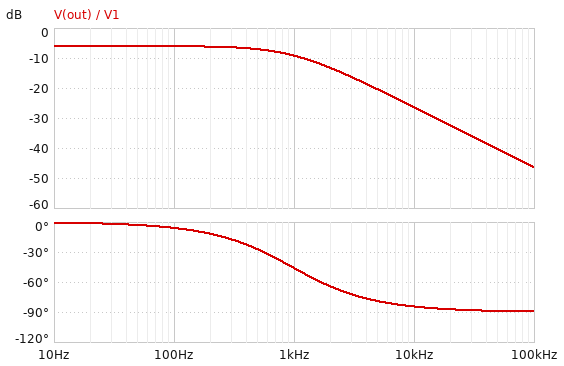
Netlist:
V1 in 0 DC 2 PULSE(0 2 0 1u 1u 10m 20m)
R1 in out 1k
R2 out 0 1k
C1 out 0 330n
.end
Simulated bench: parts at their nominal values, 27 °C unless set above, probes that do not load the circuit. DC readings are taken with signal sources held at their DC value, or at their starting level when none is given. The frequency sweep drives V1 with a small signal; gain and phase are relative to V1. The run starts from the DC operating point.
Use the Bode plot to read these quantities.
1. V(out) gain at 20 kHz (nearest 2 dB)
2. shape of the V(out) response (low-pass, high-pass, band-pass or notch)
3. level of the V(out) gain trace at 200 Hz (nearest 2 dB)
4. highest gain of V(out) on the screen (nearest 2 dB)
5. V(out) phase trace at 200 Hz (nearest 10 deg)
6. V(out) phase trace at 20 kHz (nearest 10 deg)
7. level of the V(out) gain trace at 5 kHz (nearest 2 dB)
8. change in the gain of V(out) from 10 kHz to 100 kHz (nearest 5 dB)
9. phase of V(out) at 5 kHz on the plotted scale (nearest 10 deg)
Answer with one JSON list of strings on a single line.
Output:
["-32 dB", "low-pass", "-6 dB", "-6 dB", "-10 deg", "-90 deg", "-20 dB", "-20 dB", "-80 deg"]
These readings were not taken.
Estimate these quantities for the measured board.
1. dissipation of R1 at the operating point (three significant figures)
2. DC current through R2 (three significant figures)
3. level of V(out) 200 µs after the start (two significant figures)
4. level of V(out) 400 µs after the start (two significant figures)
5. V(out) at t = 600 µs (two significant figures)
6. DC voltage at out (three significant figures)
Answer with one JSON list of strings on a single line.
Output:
["1.00 mW", "1.00 mA", "700 mV", "910 mV", "970 mV", "1.00 V"]
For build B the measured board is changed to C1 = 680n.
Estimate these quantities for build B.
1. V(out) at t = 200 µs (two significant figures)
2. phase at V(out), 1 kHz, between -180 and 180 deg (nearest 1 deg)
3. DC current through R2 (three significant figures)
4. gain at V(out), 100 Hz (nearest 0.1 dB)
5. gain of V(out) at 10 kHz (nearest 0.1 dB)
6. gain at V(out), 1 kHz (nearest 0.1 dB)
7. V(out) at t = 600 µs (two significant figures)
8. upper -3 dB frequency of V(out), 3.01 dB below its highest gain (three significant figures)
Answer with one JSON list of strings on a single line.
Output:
["440 mV", "-65 deg", "1.00 mA", "-6.2 dB", "-32.6 dB", "-13.5 dB", "830 mV", "468 Hz"]
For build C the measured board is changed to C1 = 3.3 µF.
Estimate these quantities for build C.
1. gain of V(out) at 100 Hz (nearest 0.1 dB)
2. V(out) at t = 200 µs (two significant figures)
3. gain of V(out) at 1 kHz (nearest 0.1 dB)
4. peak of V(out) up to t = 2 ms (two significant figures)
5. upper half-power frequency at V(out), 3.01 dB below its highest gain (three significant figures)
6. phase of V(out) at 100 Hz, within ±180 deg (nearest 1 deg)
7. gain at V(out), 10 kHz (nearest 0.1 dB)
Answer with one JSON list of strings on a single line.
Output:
["-9.2 dB", "110 mV", "-26.4 dB", "700 mV", "96.5 Hz", "-46 deg", "-46.3 dB"]
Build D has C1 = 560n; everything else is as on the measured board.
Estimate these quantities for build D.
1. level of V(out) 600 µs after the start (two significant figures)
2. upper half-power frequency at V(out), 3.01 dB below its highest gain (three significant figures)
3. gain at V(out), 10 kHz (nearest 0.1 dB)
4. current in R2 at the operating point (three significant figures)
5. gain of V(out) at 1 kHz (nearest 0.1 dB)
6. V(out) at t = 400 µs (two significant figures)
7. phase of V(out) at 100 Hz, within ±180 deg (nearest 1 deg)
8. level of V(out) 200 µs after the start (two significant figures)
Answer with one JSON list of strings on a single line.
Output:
["880 mV", "568 Hz", "-30.9 dB", "1.00 mA", "-12.1 dB", "760 mV", "-10 deg", "510 mV"]
